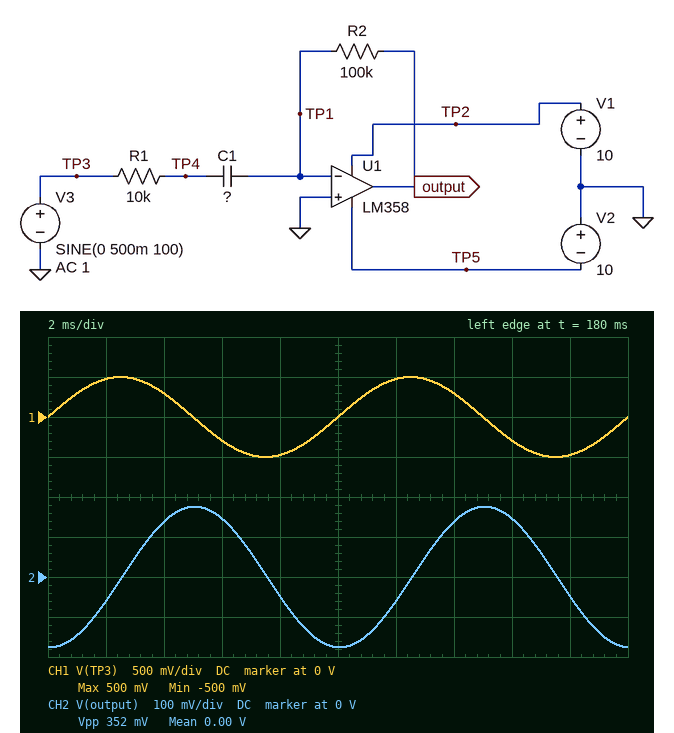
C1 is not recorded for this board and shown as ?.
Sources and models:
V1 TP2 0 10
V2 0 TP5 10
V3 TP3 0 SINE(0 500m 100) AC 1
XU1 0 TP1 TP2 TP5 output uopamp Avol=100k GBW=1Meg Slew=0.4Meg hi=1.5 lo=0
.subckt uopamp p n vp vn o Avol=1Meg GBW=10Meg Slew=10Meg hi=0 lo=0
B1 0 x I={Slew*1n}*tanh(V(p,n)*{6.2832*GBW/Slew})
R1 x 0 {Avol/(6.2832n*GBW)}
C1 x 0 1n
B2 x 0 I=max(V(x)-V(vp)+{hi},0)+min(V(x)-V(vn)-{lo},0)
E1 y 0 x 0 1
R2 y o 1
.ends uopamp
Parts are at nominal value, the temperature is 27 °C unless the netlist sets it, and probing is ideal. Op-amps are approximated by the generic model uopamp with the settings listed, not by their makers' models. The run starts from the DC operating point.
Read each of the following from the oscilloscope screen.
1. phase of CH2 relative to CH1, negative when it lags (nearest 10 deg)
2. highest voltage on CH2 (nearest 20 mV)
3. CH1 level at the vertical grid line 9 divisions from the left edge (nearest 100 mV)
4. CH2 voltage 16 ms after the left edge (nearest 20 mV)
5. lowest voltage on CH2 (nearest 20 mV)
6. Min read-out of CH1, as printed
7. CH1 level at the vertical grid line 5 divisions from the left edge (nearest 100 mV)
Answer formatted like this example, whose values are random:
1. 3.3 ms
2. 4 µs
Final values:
1. -90 deg
2. 180 mV
3. -500 mV
4. 140 mV
5. -180 mV
6. -500 mV
7. 0 V
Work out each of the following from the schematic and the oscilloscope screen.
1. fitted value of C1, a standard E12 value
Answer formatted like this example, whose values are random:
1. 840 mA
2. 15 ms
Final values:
1. 5.6 nF
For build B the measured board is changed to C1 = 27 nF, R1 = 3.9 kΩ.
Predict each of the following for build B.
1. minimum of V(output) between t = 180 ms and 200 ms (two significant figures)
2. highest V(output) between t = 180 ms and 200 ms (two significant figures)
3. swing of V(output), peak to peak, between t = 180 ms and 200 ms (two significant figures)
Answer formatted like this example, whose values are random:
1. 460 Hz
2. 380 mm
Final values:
1. -850 mV
2. 850 mV
3. 1.7 V
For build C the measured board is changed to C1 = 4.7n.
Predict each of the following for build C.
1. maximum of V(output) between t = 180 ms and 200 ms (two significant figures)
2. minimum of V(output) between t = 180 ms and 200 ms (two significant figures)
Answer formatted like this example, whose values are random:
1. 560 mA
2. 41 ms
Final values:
1. 150 mV
2. -150 mV
